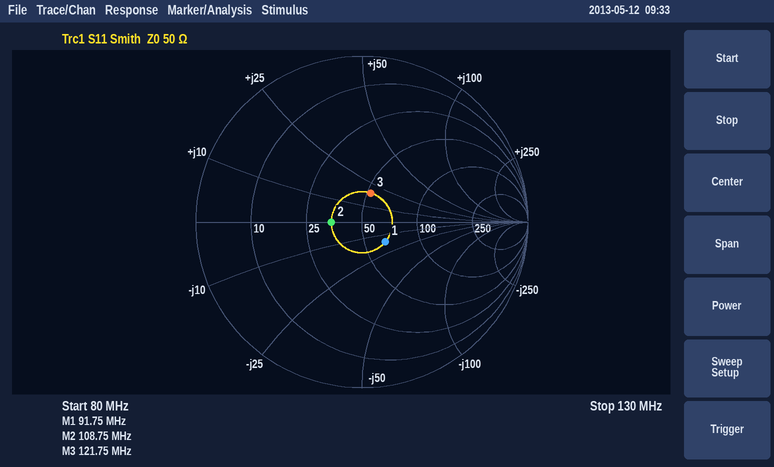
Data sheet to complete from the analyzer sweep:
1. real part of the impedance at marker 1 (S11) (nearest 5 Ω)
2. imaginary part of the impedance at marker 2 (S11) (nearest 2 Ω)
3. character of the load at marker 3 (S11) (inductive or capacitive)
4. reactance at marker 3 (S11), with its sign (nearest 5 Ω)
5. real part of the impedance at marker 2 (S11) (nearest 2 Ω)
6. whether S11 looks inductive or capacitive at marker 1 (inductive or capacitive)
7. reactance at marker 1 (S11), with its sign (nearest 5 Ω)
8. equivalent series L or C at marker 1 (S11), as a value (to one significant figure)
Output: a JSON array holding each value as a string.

["65 Ω", "0 Ω", "inductive", "+20 Ω", "34 Ω", "capacitive", "-15 Ω", "100 pF"]
